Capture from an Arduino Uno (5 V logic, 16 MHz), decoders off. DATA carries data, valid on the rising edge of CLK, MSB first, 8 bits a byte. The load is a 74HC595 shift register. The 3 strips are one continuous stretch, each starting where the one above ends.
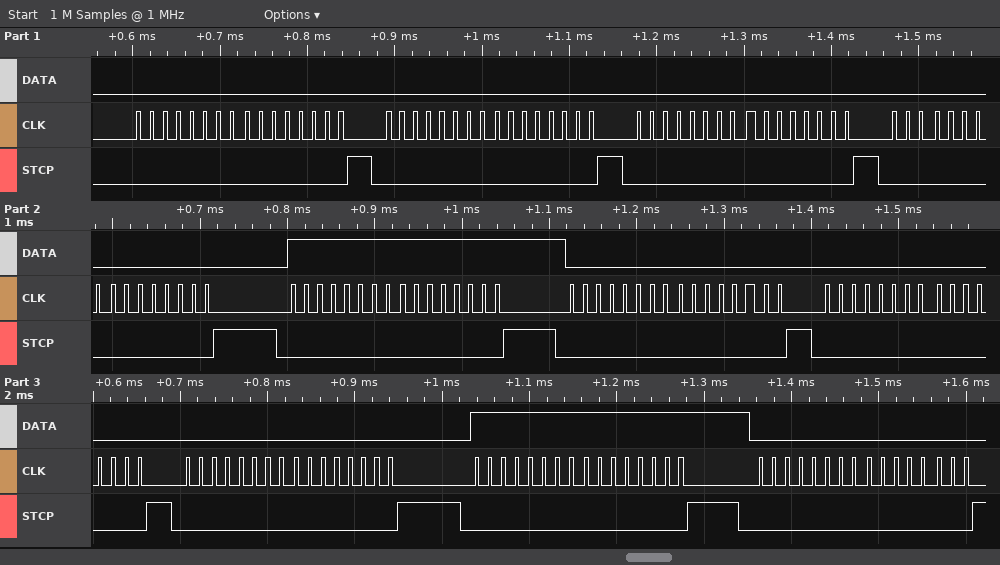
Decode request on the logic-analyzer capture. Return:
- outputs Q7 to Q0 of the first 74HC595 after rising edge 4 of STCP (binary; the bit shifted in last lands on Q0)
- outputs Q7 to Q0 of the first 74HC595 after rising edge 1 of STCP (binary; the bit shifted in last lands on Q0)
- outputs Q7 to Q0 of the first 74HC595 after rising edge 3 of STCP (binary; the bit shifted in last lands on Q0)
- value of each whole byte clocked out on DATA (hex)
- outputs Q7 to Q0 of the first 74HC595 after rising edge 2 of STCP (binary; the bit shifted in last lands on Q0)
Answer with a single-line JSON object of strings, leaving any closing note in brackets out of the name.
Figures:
{"outputs Q7 to Q0 of the first 74HC595 after rising edge 4 of STCP": "00000000", "outputs Q7 to Q0 of the first 74HC595 after rising edge 1 of STCP": "00000000", "outputs Q7 to Q0 of the first 74HC595 after rising edge 3 of STCP": "00000000", "value of each whole byte clocked out on DATA": "00 00 00 00 00 00 00 00 FF FF 00 00 00 00 00 00 FF FF 00 00", "outputs Q7 to Q0 of the first 74HC595 after rising edge 2 of STCP": "00000000"}
